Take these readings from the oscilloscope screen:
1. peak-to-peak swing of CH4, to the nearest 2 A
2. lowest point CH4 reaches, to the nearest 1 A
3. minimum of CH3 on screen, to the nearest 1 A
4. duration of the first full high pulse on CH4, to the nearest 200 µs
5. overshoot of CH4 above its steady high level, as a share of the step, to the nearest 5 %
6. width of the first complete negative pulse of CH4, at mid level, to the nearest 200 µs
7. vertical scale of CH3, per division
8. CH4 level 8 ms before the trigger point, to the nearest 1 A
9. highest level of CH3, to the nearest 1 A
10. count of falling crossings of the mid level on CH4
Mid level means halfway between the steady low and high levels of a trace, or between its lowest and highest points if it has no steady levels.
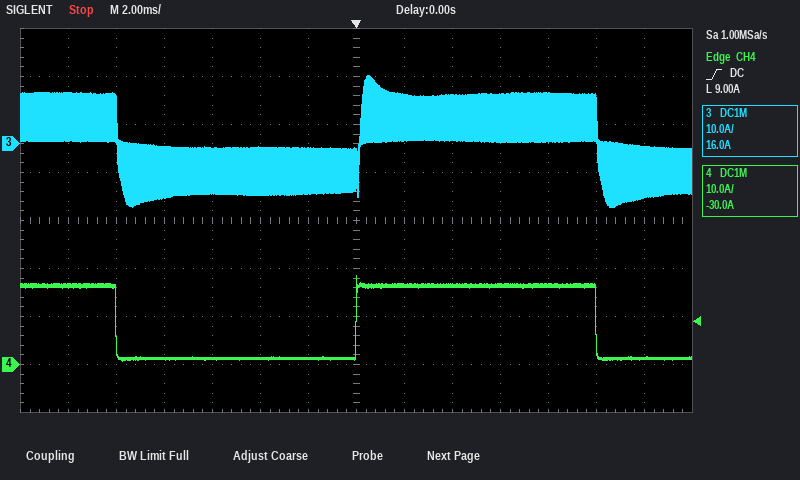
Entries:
18 A
1 A
-13 A
10.0 ms
15 %
10.0 ms
10 A
1 A
14 A
2
